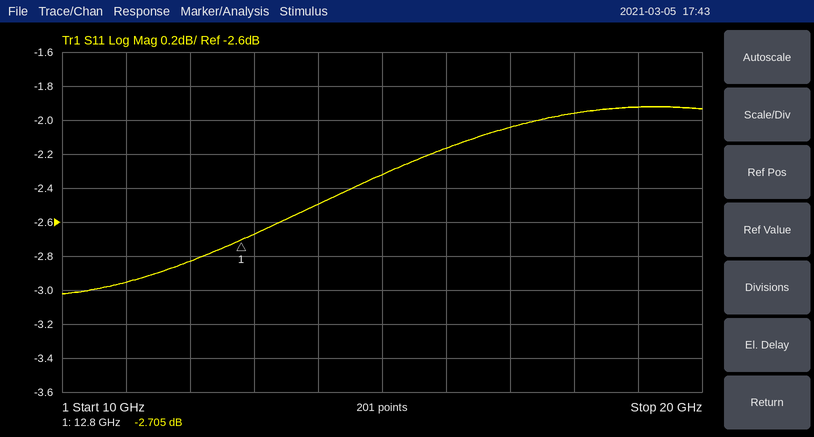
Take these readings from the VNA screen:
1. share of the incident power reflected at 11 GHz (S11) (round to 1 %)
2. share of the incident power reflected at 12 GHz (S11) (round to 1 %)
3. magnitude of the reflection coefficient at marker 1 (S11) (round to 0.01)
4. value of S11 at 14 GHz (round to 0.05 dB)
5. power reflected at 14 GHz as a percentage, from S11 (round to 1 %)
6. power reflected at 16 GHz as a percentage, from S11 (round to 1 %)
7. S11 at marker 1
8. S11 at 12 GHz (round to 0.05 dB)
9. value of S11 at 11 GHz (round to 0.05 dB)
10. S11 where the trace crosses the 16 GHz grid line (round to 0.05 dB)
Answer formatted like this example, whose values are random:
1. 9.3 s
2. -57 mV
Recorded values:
1. 51 %
2. 52 %
3. 0.73
4. -2.50 dB
5. 56 %
6. 61 %
7. -2.705 dB
8. -2.85 dB
9. -2.95 dB
10. -2.15 dB
